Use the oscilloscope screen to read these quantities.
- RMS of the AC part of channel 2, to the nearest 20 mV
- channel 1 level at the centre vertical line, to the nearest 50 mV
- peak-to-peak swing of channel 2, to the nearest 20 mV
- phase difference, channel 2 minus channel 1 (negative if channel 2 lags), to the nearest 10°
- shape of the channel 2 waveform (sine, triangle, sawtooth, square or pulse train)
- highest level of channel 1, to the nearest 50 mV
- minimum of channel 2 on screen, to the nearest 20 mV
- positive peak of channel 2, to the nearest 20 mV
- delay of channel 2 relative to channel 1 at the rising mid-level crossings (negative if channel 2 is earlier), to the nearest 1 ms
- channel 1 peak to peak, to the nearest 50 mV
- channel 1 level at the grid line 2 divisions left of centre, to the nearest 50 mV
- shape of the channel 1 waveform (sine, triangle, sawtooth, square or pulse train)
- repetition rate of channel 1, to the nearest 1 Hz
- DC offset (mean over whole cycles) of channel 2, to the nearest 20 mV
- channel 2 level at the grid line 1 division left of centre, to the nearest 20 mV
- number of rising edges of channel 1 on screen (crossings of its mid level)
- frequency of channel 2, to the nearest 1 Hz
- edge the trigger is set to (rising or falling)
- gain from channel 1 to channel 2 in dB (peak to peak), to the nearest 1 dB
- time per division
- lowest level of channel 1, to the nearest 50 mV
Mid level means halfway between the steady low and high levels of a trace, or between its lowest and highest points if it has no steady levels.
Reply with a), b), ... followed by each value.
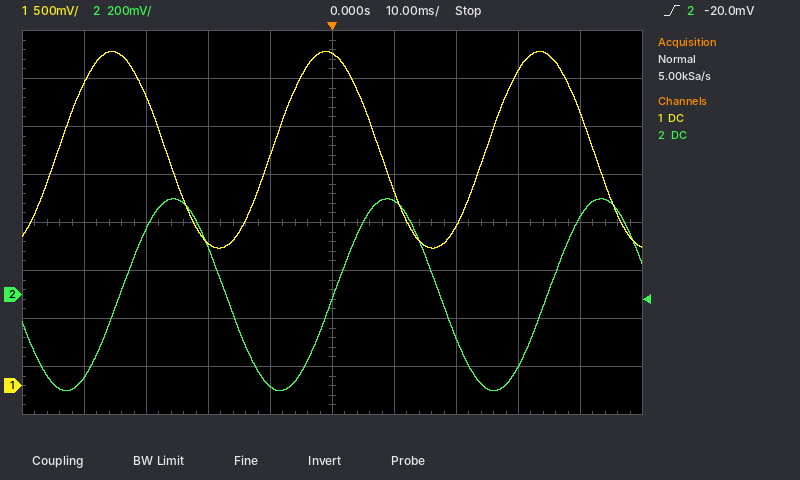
a) 280 mV
b) 3.45 V
c) 800 mV
d) -100°
e) sine
f) 3.50 V
g) -400 mV
h) 400 mV
i) +10 ms
j) 2.05 V
k) 1.50 V
l) sine
m) 29 Hz
n) 0 mV
o) -380 mV
p) 3
q) 29 Hz
r) rising
s) -8 dB
t) 10 ms
u) 1.45 V
